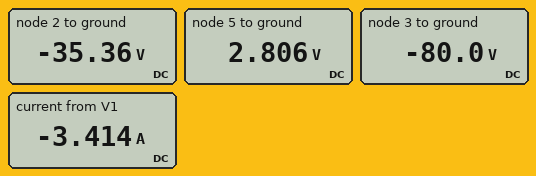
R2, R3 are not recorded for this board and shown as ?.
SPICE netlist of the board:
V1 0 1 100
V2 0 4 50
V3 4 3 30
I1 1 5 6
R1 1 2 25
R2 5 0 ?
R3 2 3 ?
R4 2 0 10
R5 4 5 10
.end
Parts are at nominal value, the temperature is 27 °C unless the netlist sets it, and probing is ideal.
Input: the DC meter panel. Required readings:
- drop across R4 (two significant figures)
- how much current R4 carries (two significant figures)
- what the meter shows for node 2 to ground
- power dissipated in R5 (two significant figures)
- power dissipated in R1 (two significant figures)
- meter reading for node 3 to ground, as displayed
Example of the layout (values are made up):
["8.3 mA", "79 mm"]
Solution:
["35 V", "3.5 A", "-35.36 V", "280 W", "170 W", "-80.0 V"]
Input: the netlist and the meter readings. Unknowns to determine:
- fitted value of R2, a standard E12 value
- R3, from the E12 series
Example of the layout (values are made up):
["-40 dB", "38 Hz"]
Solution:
["3.9 Ω", "47 Ω"]
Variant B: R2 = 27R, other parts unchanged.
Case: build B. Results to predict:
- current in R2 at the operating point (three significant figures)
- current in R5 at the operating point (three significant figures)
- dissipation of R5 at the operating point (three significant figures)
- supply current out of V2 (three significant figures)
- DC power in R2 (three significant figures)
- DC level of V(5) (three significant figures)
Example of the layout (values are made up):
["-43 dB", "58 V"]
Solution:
["270 mA", "5.73 A", "328 W", "6.68 A", "1.97 W", "7.30 V"]
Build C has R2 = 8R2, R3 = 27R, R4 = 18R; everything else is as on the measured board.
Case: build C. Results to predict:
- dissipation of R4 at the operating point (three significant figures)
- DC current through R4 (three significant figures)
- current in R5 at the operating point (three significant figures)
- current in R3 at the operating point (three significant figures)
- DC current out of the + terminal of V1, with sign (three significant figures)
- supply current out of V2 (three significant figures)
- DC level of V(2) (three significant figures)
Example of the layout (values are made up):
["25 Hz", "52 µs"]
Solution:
["153 W", "2.92 A", "5.45 A", "1.02 A", "-4.10 A", "6.47 A", "-52.5 V"]
